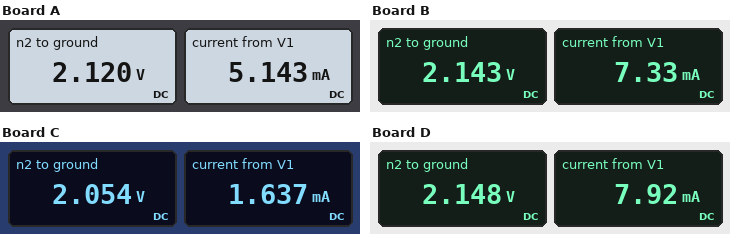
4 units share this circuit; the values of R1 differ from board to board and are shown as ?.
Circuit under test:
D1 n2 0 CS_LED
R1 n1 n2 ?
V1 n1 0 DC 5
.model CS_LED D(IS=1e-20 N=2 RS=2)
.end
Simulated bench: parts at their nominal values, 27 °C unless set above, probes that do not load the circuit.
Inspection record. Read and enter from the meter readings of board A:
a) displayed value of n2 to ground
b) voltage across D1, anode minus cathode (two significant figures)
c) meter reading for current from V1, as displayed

2.120 V
2.1 V
5.143 mA
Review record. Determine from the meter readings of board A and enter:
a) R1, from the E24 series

560 Ω
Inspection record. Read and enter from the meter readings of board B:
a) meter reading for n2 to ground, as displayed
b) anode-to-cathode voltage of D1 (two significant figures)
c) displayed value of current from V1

2.143 V
2.1 V
7.33 mA
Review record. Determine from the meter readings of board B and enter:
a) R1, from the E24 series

390 Ω
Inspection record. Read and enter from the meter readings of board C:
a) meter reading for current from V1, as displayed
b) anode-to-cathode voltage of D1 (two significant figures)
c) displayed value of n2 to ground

1.637 mA
2.1 V
2.054 V
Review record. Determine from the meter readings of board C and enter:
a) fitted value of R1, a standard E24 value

1.8 kΩ
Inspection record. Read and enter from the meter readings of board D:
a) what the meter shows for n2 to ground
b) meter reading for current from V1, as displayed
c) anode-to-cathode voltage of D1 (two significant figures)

2.148 V
7.92 mA
2.1 V
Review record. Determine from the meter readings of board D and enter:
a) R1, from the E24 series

360 Ω
